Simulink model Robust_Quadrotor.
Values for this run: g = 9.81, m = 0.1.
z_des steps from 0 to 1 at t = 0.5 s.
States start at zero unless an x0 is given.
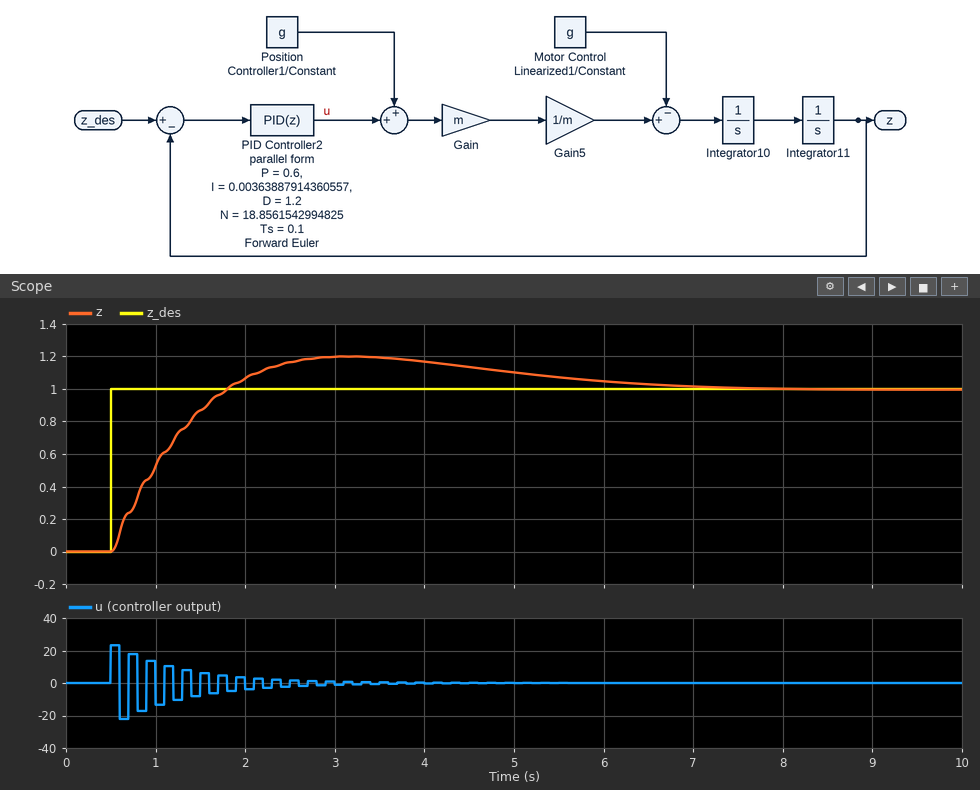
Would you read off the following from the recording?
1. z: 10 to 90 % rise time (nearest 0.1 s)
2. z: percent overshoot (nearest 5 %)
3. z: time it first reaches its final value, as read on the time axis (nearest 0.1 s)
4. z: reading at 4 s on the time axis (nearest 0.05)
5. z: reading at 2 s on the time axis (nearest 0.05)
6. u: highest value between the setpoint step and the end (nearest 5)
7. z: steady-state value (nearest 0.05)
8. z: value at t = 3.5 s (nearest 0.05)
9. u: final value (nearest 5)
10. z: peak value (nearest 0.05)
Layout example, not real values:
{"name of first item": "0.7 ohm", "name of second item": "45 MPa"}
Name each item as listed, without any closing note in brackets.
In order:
{"z: 10 to 90 % rise time": "1.0 s", "z: percent overshoot": "20 %", "z: time it first reaches its final value, as read on the time axis": "1.8 s", "z: reading at 4 s on the time axis": "1.15", "z: reading at 2 s on the time axis": "1.05", "u: highest value between the setpoint step and the end": "25", "z: steady-state value": "1.00", "z: value at t = 3.5 s": "1.20", "u: final value": "0", "z: peak value": "1.20"}
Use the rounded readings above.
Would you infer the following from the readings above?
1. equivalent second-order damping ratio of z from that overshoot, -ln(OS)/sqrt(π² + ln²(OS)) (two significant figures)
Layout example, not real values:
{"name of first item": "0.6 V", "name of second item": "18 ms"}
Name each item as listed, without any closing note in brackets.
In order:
{"equivalent second-order damping ratio of z from that overshoot, -ln(OS)/sqrt(π² + ln²(OS))": "0.46"}
